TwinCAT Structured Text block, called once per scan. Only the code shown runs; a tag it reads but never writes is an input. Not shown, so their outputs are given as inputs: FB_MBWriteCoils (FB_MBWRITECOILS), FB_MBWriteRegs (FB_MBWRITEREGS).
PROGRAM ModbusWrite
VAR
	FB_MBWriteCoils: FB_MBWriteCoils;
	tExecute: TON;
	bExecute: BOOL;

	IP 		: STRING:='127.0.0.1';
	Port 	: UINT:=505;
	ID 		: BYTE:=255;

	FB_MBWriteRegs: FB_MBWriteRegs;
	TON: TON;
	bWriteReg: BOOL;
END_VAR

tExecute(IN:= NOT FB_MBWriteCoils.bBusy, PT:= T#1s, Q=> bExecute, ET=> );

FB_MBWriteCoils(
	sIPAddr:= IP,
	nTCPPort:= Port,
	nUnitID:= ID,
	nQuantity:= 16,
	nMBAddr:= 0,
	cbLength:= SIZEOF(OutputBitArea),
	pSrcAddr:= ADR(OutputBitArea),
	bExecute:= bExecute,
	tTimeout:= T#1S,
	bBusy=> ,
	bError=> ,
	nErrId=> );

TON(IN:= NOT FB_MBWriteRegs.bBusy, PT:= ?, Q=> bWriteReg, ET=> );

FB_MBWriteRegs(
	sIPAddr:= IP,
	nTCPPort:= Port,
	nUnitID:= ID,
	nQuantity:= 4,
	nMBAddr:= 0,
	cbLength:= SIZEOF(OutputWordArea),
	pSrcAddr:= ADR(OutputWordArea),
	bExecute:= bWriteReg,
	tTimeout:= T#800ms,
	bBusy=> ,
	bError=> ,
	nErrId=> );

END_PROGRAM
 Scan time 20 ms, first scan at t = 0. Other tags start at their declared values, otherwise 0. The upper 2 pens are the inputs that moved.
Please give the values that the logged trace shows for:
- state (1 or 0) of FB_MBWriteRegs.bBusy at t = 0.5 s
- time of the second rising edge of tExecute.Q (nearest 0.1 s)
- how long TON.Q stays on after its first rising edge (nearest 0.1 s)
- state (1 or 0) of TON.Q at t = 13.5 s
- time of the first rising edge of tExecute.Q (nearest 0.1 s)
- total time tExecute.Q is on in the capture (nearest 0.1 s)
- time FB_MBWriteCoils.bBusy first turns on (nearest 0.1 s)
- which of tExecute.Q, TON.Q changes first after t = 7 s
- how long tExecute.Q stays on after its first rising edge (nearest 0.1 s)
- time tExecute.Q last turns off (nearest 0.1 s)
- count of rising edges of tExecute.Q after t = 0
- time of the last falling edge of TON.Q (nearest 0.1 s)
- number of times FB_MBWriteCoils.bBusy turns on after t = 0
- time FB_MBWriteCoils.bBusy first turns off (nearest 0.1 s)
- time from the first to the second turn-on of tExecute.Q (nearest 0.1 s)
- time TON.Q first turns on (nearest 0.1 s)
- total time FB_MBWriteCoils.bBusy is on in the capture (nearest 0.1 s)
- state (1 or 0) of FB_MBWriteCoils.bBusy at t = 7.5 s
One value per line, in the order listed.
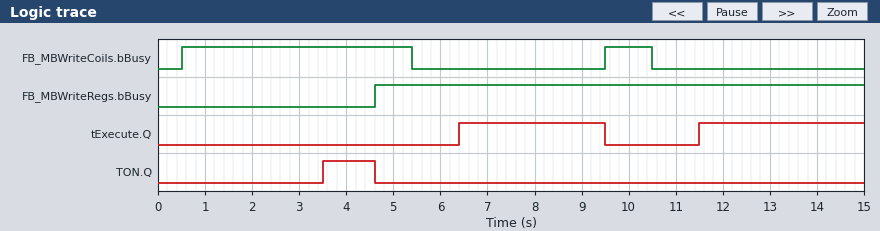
0
11.5 s
1.1 s
0
6.4 s
6.6 s
0.5 s
tExecute.Q
3.1 s
9.5 s
2
4.6 s
2
5.4 s
5.1 s
3.5 s
5.9 s
0
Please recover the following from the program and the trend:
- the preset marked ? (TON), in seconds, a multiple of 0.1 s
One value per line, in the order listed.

3.5 s
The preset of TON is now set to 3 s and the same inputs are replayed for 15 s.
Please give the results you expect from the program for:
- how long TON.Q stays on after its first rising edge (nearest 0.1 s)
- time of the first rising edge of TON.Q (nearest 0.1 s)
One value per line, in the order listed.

1.6 s
3.0 s
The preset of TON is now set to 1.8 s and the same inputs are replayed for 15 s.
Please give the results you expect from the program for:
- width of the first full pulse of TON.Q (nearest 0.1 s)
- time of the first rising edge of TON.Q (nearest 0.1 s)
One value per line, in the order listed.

2.8 s
1.8 s
